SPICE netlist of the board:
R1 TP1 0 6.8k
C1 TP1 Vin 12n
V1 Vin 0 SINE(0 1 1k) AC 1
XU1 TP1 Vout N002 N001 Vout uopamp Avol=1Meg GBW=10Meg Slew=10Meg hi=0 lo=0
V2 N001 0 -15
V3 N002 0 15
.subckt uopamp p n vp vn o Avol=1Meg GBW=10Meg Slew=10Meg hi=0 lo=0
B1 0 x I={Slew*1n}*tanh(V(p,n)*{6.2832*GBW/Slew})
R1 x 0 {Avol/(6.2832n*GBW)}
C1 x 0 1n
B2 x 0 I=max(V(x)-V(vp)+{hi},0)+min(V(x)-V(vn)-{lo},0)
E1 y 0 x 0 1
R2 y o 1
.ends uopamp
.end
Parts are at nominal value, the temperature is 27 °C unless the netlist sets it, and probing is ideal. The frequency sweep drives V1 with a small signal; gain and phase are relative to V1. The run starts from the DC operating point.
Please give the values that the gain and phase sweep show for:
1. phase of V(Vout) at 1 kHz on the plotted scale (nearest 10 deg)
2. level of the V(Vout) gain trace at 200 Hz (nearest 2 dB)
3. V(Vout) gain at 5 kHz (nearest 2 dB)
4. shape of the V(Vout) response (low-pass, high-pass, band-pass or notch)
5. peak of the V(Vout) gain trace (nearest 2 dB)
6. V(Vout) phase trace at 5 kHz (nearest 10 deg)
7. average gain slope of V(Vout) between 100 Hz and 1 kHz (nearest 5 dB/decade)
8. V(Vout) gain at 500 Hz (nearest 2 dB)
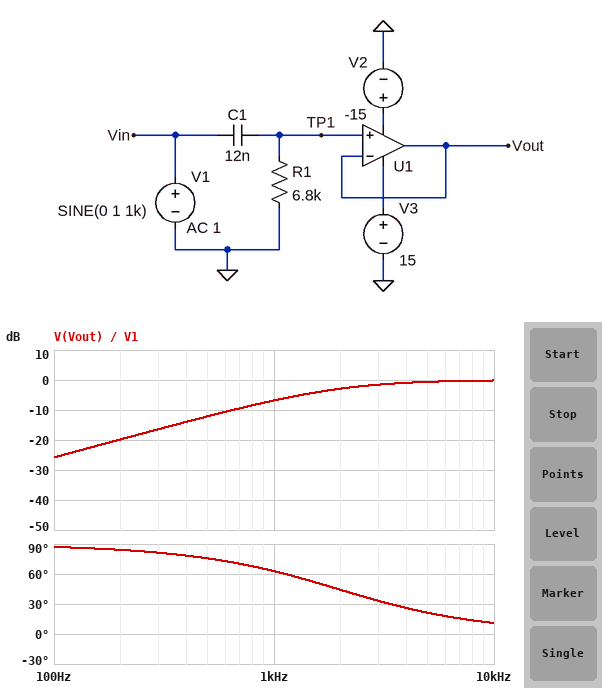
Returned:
60 deg
-20 dB
0 dB
high-pass
0 dB
20 deg
20 dB/decade
-12 dB
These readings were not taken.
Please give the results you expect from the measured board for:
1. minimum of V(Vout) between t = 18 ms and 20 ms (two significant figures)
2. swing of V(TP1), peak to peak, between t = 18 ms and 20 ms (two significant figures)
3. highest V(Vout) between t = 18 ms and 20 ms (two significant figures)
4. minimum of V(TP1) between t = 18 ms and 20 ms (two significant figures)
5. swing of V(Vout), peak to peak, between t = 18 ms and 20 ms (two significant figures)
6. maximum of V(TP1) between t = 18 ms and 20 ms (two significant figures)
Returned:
-460 mV
910 mV
460 mV
-460 mV
910 mV
460 mV
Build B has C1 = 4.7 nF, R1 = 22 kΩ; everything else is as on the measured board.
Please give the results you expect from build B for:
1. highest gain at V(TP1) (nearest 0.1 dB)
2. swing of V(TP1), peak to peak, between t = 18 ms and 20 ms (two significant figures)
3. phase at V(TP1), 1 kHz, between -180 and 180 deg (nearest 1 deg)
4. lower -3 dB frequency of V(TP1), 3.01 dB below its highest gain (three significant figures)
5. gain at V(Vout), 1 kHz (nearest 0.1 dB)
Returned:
0 dB
1.1 V
57 deg
1.54 kHz
-5.3 dB
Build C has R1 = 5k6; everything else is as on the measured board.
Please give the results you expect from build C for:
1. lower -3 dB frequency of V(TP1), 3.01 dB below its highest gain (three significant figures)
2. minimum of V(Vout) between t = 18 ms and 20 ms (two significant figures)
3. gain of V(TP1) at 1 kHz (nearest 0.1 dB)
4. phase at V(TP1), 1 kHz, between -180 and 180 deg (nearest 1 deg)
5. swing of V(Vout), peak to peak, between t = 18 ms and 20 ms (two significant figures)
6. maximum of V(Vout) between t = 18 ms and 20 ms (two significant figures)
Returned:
2.37 kHz
-390 mV
-8.2 dB
67 deg
780 mV
390 mV
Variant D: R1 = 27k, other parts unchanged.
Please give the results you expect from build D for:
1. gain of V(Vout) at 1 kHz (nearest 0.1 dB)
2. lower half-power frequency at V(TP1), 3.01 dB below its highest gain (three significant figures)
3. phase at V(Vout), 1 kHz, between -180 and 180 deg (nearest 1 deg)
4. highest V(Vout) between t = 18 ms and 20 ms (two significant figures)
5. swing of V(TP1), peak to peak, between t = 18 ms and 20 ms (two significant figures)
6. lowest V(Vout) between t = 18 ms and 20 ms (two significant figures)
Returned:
-0.9 dB
491 Hz
26 deg
900 mV
1.8 V
-900 mV
